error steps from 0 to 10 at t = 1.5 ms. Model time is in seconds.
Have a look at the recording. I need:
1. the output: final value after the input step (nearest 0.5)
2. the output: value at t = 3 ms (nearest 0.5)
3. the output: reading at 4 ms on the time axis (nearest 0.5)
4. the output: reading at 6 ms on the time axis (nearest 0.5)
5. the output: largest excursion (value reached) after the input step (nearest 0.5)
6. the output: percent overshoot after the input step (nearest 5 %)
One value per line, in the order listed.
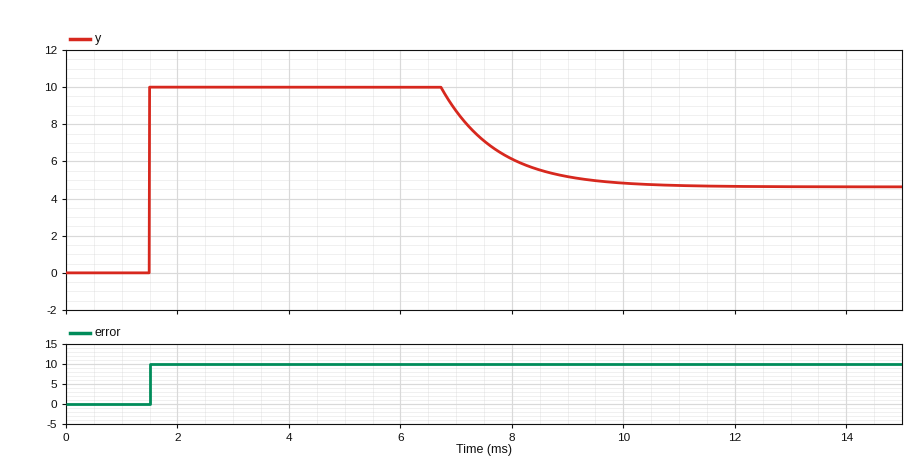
4.5
10.0
10.0
10.0
10.0
115 %
